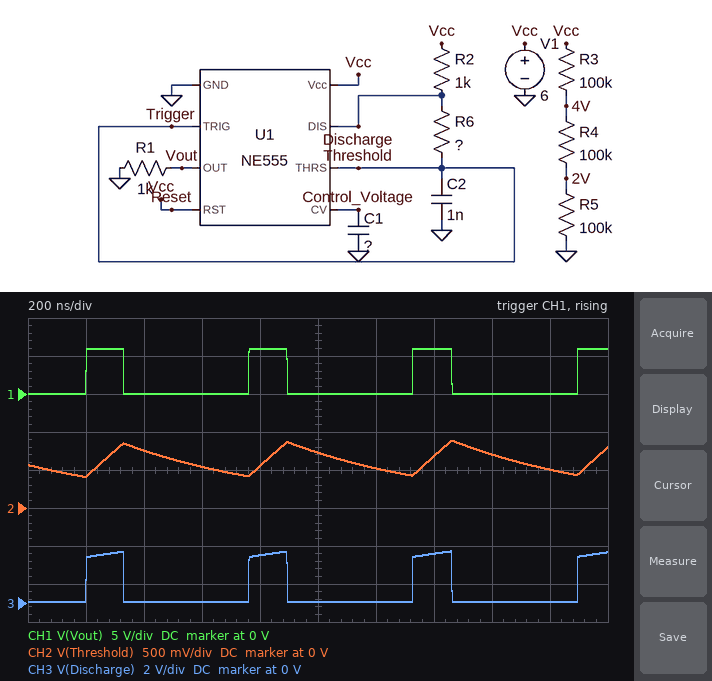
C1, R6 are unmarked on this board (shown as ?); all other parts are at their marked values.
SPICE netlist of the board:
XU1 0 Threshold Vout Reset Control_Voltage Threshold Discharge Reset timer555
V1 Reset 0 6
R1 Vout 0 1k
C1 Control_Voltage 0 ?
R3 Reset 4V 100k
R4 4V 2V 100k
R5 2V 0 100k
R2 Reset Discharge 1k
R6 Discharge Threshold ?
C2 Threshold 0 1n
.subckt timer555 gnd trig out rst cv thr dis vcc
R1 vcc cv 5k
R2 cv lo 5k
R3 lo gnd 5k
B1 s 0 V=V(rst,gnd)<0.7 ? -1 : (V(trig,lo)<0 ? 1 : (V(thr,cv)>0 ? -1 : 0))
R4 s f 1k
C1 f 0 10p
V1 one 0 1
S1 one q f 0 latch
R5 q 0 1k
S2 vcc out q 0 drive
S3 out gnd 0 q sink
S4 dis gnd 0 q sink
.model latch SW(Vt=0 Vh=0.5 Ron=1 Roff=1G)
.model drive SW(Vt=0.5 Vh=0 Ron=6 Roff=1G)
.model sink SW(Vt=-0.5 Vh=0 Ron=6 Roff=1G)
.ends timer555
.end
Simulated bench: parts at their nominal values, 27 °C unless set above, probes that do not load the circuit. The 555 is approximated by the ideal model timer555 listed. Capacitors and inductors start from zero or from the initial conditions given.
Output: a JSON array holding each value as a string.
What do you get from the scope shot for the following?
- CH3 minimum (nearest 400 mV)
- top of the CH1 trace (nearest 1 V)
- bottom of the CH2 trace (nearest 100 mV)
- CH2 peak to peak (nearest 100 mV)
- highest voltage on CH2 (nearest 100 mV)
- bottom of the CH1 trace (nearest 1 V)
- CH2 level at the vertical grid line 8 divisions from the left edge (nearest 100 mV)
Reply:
["0 V", "6 V", "400 mV", "500 mV", "900 mV", "0 V", "700 mV"]
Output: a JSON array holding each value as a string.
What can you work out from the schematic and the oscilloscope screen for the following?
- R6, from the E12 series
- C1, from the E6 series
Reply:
["560 Ω", "33 nF"]
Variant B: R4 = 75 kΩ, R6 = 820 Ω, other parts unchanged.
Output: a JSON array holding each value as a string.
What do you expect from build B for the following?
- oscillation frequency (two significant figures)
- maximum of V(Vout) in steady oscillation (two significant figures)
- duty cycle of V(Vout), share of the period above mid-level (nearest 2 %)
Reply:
["1.3 MHz", "6.0 V", "20 %"]
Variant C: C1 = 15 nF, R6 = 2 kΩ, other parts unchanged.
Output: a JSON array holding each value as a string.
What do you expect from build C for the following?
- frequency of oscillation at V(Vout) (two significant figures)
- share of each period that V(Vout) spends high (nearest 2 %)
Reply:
["520 kHz", "28 %"]
